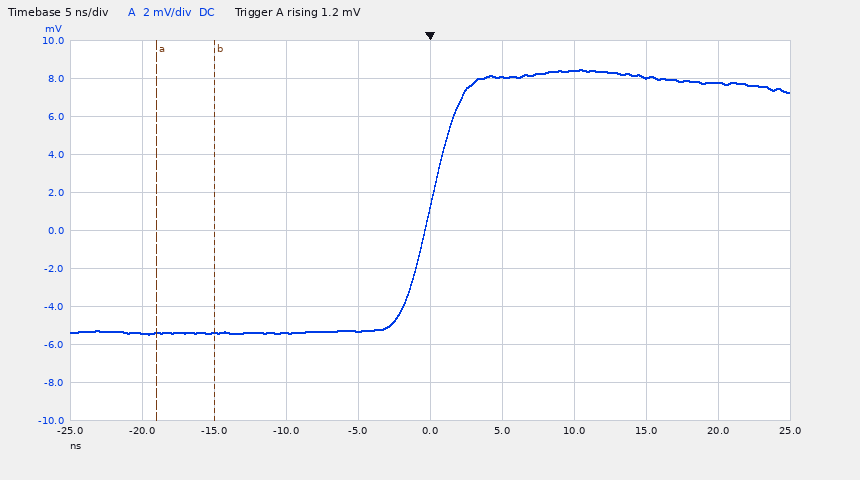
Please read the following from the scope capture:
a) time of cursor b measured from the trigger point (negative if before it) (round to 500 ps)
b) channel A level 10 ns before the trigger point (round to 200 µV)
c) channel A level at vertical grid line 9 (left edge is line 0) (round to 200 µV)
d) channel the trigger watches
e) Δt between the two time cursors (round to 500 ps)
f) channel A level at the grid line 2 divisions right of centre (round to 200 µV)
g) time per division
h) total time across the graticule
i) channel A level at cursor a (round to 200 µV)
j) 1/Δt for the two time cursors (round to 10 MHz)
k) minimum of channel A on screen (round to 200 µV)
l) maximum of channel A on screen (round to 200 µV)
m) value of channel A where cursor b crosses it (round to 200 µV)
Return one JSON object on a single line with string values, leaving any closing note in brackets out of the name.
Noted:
{"time of cursor b measured from the trigger point (negative if before it)": "-15.0 ns", "channel A level 10 ns before the trigger point": "-5.4 mV", "channel A level at vertical grid line 9 (left edge is line 0)": "7.8 mV", "channel the trigger watches": "channel A", "Δt between the two time cursors": "4.0 ns", "channel A level at the grid line 2 divisions right of centre": "8.4 mV", "time per division": "5 ns", "total time across the graticule": "50 ns", "channel A level at cursor a": "-5.4 mV", "1/Δt for the two time cursors": "250 MHz", "minimum of channel A on screen": "-5.4 mV", "maximum of channel A on screen": "8.4 mV", "value of channel A where cursor b crosses it": "-5.4 mV"}
